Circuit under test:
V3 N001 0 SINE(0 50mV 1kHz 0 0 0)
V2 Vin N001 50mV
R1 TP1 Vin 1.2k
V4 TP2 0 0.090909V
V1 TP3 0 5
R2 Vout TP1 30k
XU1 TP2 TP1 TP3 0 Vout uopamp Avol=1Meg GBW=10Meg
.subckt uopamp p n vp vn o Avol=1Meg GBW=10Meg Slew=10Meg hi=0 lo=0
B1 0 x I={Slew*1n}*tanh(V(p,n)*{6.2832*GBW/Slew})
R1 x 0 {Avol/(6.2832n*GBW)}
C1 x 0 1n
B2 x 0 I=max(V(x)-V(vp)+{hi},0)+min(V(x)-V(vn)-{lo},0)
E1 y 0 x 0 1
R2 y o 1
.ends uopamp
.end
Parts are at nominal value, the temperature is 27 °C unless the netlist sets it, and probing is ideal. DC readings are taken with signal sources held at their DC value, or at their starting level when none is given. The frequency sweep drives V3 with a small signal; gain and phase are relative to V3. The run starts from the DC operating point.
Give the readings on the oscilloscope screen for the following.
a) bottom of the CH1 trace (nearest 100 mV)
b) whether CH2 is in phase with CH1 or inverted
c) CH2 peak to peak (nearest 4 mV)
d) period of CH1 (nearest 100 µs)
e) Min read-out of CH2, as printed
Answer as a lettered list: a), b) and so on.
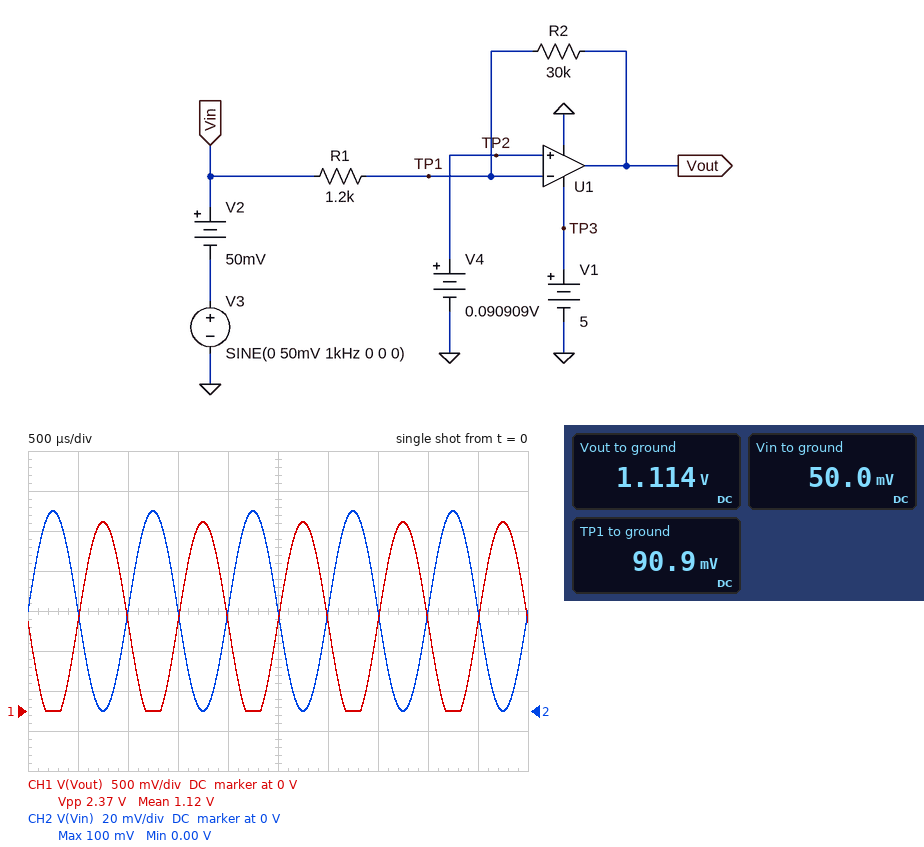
a) 0 V
b) inverted
c) 100 mV
d) 1.0 ms
e) 0.00 V
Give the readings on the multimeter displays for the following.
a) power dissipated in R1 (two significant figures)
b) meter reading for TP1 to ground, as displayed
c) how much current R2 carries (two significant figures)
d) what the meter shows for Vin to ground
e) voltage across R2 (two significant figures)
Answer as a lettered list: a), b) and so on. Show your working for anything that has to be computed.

a) (90.9 mV - 50 mV)^2 / 1.2 kΩ = 1.4 µW
b) 90.9 mV
c) (1.114 V - 90.9 mV) / 30 kΩ = 34 µA
d) 50.0 mV
e) 1.114 V - 90.9 mV = 1.0 V
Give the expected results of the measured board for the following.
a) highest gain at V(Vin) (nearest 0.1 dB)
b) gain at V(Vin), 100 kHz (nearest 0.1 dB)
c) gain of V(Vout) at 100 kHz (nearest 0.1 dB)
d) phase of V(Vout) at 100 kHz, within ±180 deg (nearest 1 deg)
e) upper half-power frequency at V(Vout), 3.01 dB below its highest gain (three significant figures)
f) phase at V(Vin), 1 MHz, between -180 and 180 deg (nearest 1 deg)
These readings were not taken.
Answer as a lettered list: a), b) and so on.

a) 0 dB
b) 0 dB
c) 27.7 dB
d) 165 deg
e) 385 kHz
f) 0 deg
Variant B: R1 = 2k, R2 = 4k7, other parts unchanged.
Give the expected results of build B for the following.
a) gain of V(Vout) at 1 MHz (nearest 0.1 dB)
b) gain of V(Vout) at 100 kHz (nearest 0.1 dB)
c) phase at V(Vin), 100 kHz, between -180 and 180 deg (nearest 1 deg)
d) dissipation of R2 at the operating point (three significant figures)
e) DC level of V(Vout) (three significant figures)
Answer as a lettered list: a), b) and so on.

a) 7.0 dB
b) 7.4 dB
c) 0 deg
d) 1.97 µW
e) 187 mV
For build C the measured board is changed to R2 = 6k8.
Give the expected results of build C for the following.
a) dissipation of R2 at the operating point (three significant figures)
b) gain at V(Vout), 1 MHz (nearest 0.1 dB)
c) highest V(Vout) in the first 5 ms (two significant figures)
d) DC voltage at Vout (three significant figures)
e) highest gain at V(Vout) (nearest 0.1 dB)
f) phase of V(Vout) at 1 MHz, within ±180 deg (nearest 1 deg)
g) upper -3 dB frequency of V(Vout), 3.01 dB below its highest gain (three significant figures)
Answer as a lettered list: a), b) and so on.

a) 7.90 µW
b) 13.5 dB
c) 610 mV
d) 323 mV
e) 15.1 dB
f) 146 deg
g) 1.50 MHz
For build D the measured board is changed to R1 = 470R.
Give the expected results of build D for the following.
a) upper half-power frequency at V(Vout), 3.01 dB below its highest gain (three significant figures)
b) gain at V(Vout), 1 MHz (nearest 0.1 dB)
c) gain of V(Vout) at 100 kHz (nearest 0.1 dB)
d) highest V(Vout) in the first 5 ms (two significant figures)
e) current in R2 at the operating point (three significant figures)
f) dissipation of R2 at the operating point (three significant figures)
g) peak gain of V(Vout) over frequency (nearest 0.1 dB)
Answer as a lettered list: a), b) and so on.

a) 154 kHz
b) 19.8 dB
c) 34.6 dB
d) 5.0 V
e) 87.0 µA
f) 227 µW
g) 36.1 dB
